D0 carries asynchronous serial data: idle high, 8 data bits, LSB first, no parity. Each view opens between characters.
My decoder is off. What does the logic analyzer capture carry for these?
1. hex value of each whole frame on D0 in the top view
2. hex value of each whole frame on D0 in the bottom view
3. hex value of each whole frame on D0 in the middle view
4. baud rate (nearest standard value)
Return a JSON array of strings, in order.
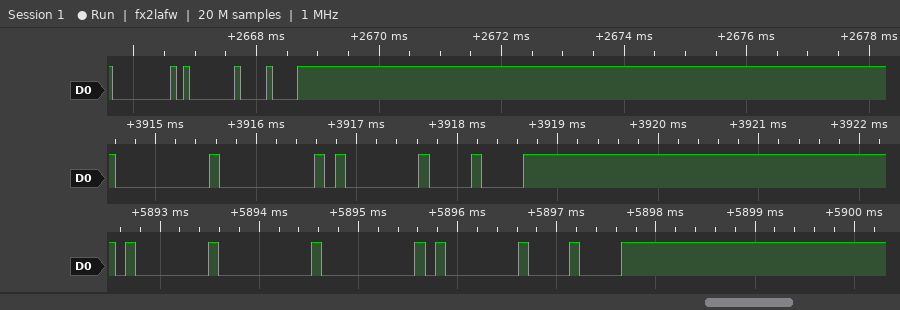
["00, 01, 08", "01, 00, 00, 01, 08", "00, 00, 01, 08", "9600 baud"]
